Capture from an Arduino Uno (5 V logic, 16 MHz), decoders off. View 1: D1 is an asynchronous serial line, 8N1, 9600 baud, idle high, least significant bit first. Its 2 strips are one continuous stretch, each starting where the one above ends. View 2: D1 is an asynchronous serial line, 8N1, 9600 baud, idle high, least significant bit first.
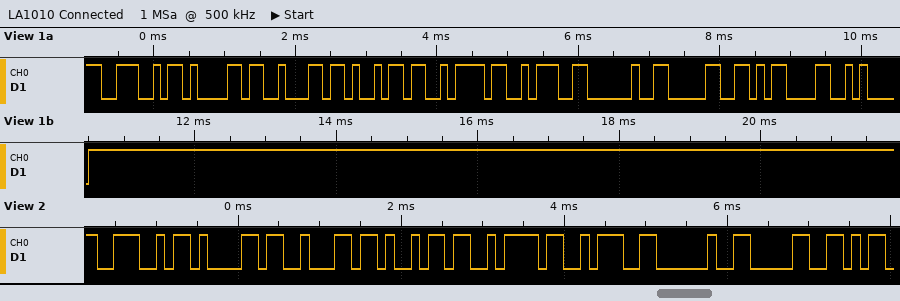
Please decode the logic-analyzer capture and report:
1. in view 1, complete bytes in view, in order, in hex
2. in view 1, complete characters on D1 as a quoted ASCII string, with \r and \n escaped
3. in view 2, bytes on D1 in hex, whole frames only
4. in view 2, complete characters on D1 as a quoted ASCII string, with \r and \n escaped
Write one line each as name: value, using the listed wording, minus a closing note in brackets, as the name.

in view 1, complete bytes in view, in order, in hex: 4E 61 62 69 7A 3A 20 30 0D 0A
in view 1, complete characters on D1 as a quoted ASCII string, with \r and \n escaped: "Nabiz: 0\r\n"
in view 2, bytes on D1 in hex, whole frames only: 4E 61 62 69 7A 3A 20 30
in view 2, complete characters on D1 as a quoted ASCII string, with \r and \n escaped: "Nabiz: 0"
